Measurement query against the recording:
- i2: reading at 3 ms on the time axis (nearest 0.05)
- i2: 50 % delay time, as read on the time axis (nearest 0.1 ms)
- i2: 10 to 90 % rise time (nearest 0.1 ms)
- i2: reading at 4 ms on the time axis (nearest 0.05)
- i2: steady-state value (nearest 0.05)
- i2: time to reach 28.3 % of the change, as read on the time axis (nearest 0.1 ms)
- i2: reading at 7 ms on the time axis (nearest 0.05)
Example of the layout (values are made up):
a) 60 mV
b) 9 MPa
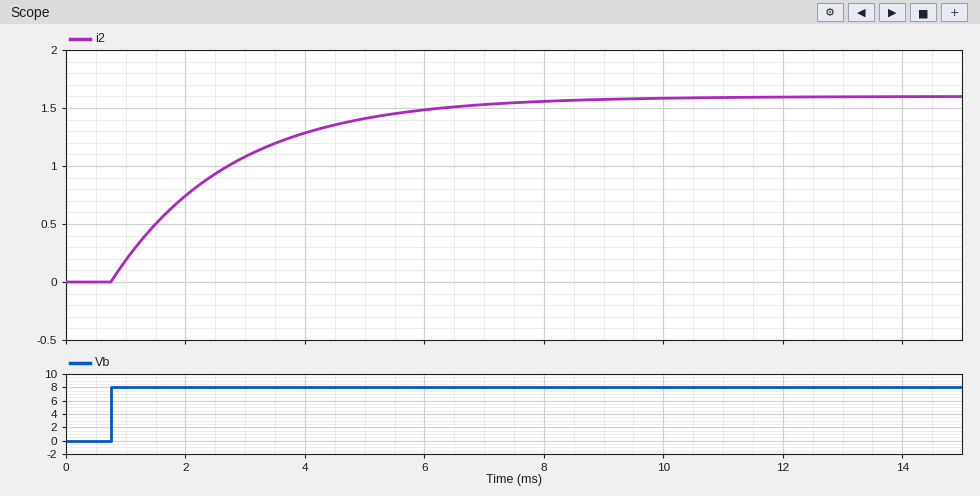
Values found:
a) 1.10
b) 2.1 ms
c) 4.4 ms
d) 1.30
e) 1.60
f) 1.4 ms
g) 1.55
